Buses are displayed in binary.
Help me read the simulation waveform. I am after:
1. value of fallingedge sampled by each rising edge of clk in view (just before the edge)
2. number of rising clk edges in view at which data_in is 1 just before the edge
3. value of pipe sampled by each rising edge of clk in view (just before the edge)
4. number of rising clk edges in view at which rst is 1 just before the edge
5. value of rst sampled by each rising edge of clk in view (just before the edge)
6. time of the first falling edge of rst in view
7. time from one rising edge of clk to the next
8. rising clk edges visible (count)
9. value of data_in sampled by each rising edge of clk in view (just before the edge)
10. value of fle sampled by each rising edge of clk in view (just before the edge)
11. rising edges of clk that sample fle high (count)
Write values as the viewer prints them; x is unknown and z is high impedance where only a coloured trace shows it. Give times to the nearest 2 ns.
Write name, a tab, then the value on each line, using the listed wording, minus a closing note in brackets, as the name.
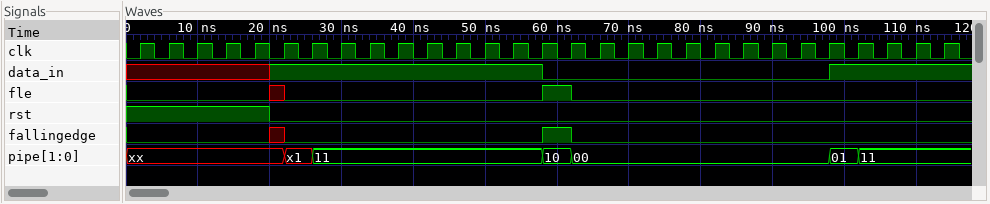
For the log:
value of fallingedge sampled by each rising edge of clk in view	0 0 0 0 0 x 0 0 0 0 0 0 0 0 0 1 0 0 0 0 0 0 0 0 0 0 0 0 0
number of rising clk edges in view at which data_in is 1 just before the edge	14
value of pipe sampled by each rising edge of clk in view	xx, xx, xx, xx, xx, xx, x1, 11, 11, 11, 11, 11, 11, 11, 11, 10, 00, 00, 00, 00, 00, 00, 00, 00, 00, 01, 11, 11, 11
number of rising clk edges in view at which rst is 1 just before the edge	5
value of rst sampled by each rising edge of clk in view	1 1 1 1 1 0 0 0 0 0 0 0 0 0 0 0 0 0 0 0 0 0 0 0 0 0 0 0 0
time of the first falling edge of rst in view	20 ns
time from one rising edge of clk to the next	4 ns
rising clk edges visible	29
value of data_in sampled by each rising edge of clk in view	x x x x x 1 1 1 1 1 1 1 1 1 1 0 0 0 0 0 0 0 0 0 0 1 1 1 1
value of fle sampled by each rising edge of clk in view	0 0 0 0 0 x 0 0 0 0 0 0 0 0 0 1 0 0 0 0 0 0 0 0 0 0 0 0 0
rising edges of clk that sample fle high	1
